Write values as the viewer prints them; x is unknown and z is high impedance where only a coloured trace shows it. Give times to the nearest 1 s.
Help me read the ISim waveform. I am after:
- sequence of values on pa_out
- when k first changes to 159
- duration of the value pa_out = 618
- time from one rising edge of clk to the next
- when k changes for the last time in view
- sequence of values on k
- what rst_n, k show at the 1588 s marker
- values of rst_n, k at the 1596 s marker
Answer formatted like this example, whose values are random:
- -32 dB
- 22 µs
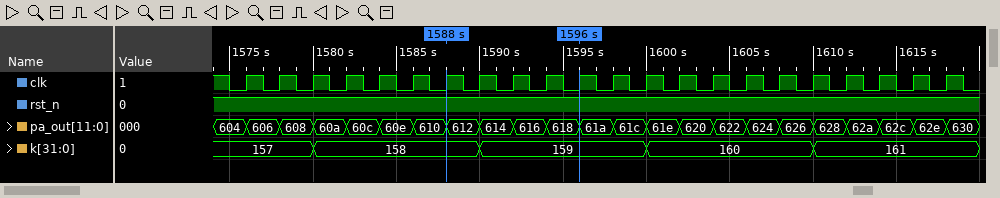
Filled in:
- 604, 606, 608, 60a, 60c, 60e, 610, 612, 614, 616, 618, 61a, 61c, 61e, 620, 622, 624, 626, 628, 62a, 62c, 62e, 630
- 1590 s
- 2 s
- 2 s
- 1610 s
- 157, 158, 159, 160, 161
- rst_n=1, k=158
- rst_n=1, k=159
